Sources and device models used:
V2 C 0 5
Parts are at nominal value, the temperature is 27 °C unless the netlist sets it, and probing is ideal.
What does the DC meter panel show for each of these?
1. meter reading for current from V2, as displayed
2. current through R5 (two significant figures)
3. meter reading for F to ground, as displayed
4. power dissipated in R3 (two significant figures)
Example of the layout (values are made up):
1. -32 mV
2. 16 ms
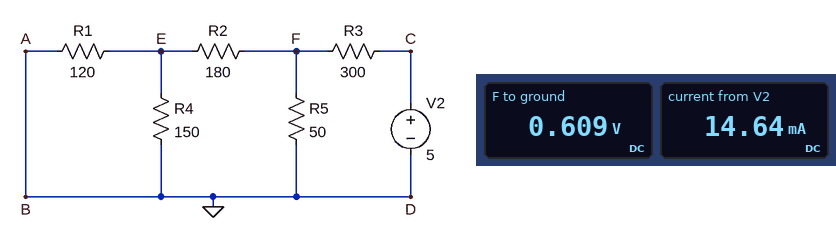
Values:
1. 14.64 mA
2. 12 mA
3. 0.609 V
4. 64 mW
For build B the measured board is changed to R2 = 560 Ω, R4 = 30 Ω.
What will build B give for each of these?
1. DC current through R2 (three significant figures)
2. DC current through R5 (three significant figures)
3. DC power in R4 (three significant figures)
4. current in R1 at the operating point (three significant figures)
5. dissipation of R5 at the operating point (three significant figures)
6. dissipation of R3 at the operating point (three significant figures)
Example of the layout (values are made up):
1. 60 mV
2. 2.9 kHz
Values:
1. 1.14 mA
2. 13.3 mA
3. 24.9 µW
4. 228 µA
5. 8.86 mW
6. 62.6 mW
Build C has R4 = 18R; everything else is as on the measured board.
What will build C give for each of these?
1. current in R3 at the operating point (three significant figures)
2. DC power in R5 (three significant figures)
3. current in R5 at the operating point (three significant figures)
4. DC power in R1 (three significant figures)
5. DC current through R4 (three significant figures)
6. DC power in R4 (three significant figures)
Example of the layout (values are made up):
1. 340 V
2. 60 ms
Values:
1. 14.7 mA
2. 6.87 mW
3. 11.7 mA
4. 18.3 µW
5. 2.60 mA
6. 122 µW
